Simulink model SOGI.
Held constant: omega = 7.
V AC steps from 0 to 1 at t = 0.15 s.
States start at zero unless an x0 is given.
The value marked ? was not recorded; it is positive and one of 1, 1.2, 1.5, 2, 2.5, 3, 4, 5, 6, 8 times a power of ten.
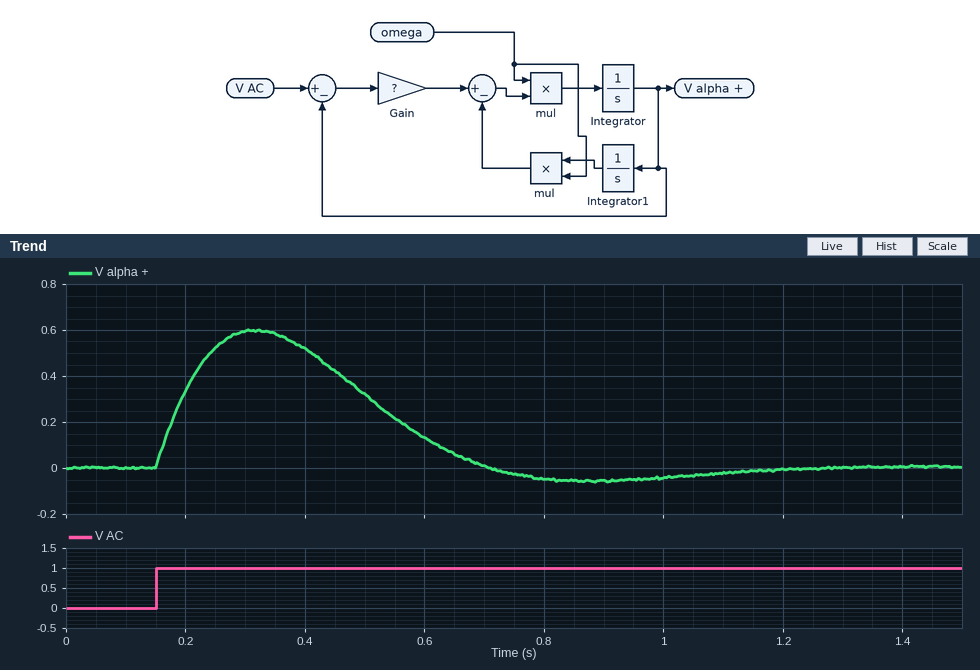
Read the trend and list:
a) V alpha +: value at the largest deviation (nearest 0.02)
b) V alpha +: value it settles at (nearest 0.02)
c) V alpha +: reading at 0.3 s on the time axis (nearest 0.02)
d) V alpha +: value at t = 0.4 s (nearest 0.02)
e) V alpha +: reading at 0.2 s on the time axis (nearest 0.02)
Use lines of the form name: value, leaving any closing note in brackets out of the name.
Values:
V alpha +: value at the largest deviation: 0.60
V alpha +: value it settles at: 0.00
V alpha +: reading at 0.3 s on the time axis: 0.60
V alpha +: value at t = 0.4 s: 0.52
V alpha +: reading at 0.2 s on the time axis: 0.34
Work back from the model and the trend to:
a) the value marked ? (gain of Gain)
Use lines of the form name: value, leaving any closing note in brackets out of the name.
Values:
the value marked ?: 1.2
